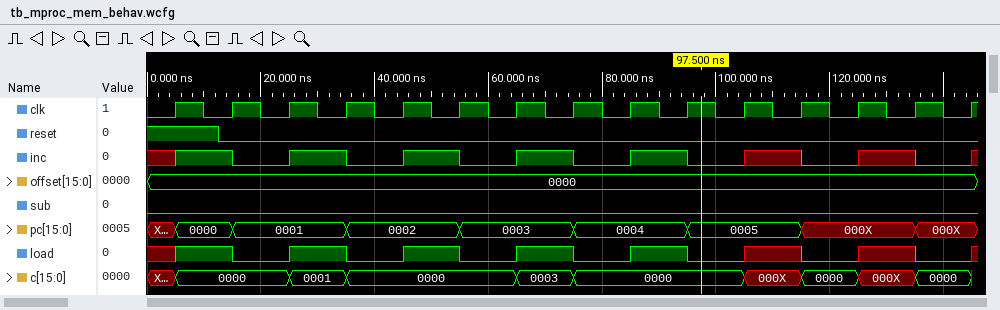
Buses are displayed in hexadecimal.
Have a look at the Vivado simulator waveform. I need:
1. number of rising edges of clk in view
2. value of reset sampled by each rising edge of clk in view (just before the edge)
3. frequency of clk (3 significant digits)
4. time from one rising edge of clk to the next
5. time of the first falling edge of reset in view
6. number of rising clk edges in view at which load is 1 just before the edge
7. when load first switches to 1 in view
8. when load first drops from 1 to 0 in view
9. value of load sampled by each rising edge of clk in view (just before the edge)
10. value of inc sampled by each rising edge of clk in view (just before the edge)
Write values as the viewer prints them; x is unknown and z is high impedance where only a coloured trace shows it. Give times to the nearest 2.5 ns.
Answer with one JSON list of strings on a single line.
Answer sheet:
["15", "1 0 0 0 0 0 0 0 0 0 0 0 0 0 0", "100 MHz", "10 ns", "12.5 ns", "5", "5 ns", "15 ns", "x 1 0 1 0 1 0 1 0 1 0 x 0 x 0", "x 1 0 1 0 1 0 1 0 1 0 x 0 x 0"]
